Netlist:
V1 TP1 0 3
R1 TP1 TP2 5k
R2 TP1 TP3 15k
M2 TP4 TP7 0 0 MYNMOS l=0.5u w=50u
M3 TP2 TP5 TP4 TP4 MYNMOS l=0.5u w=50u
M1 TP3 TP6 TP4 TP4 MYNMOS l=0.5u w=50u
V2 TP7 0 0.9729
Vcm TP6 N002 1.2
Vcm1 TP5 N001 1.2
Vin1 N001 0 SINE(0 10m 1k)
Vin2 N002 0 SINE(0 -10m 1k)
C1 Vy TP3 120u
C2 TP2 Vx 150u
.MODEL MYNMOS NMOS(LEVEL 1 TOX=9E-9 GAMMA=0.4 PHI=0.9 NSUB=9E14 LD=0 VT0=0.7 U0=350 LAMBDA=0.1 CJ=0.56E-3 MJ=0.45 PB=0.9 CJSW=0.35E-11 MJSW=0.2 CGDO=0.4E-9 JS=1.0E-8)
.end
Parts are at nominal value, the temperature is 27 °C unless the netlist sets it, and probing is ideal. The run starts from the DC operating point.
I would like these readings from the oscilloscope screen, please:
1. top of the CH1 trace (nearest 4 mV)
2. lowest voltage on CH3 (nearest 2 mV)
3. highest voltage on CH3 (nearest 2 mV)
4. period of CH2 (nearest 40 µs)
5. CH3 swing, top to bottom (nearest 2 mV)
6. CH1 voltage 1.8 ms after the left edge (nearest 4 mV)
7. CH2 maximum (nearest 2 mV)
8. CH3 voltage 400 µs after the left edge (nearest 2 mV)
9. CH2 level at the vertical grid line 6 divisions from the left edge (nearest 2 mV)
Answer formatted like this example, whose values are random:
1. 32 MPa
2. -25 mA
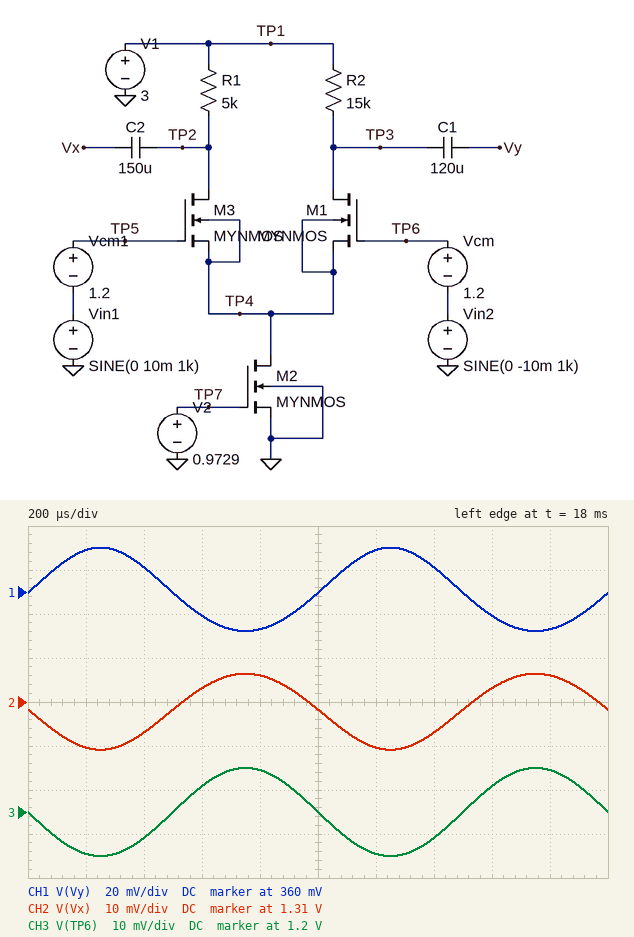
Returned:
1. 380 mV
2. 1.190 V
3. 1.210 V
4. 1.00 ms
5. 20 mV
6. 344 mV
7. 1.316 V
8. 1.194 V
9. 1.300 V
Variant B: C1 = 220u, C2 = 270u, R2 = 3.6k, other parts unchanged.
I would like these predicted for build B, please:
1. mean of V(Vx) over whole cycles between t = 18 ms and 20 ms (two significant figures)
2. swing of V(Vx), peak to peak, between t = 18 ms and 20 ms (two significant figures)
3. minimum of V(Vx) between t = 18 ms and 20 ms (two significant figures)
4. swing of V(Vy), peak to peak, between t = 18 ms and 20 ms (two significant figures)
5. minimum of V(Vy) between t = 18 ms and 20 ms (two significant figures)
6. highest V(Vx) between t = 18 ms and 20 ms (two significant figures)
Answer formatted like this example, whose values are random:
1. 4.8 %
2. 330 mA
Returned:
1. 1.7 V
2. 260 mV
3. 1.6 V
4. 190 mV
5. 2.0 V
6. 1.9 V
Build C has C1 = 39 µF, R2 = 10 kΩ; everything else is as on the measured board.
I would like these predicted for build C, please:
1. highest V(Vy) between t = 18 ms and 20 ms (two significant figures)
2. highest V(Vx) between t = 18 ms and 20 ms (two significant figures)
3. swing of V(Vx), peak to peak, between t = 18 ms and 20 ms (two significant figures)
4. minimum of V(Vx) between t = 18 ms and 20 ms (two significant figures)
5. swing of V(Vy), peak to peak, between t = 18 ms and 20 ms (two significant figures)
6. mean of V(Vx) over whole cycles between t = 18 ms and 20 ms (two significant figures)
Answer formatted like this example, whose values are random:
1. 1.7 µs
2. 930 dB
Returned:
1. 780 mV
2. 1.7 V
3. 170 mV
4. 1.5 V
5. 340 mV
6. 1.6 V
